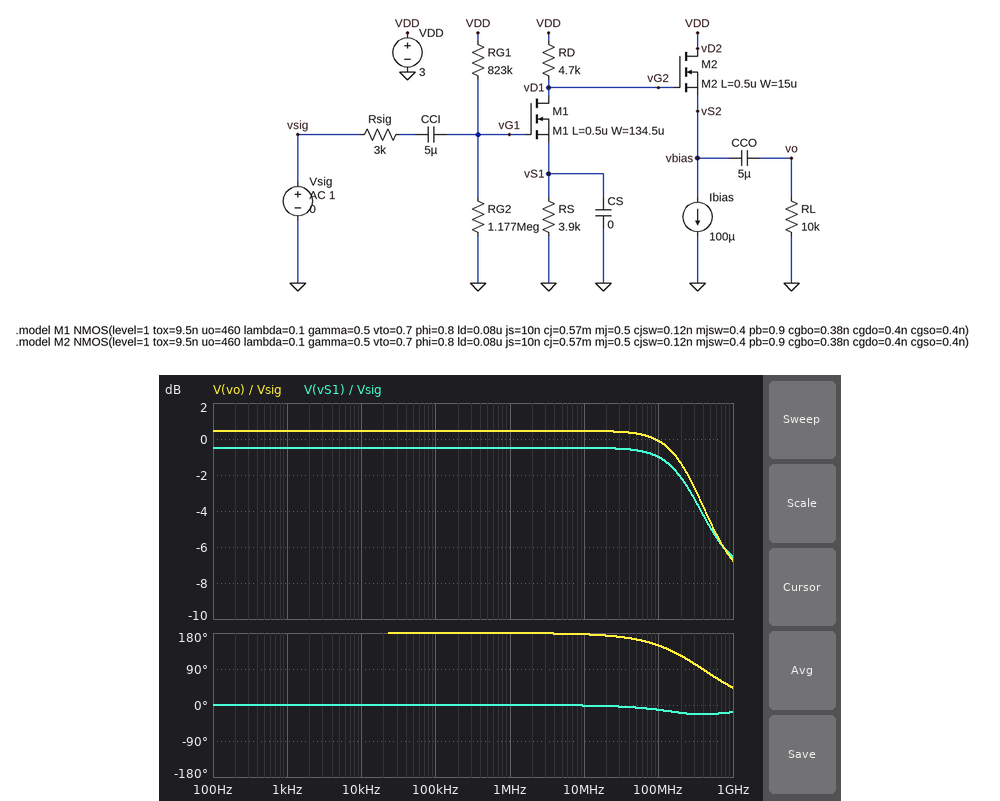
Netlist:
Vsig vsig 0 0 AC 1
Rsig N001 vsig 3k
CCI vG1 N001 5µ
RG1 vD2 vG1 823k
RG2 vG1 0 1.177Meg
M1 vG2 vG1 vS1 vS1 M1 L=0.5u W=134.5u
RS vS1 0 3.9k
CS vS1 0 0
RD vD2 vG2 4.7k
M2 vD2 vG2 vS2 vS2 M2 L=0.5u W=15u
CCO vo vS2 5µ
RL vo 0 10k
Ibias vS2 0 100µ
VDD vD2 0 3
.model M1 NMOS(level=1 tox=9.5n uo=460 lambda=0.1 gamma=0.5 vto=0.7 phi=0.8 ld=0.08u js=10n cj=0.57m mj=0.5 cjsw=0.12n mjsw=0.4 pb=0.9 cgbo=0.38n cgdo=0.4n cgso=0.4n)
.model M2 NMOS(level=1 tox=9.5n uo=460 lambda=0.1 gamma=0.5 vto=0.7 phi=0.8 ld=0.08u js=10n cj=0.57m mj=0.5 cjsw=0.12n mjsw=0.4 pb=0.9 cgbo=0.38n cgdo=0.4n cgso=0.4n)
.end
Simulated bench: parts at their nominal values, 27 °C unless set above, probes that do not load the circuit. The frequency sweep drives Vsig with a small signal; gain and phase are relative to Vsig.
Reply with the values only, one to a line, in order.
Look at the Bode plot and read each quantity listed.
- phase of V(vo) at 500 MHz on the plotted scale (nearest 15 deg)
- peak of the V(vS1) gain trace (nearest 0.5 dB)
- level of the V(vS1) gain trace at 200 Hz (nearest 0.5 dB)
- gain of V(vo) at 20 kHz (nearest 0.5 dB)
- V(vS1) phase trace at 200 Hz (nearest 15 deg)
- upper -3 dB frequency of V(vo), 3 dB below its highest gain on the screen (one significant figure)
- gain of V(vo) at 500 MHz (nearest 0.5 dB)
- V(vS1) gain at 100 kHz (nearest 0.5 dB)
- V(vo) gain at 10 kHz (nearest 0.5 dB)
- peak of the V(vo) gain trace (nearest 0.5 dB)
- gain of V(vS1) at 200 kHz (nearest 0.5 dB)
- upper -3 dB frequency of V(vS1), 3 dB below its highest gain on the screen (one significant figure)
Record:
75 deg
-0.5 dB
-0.5 dB
0.5 dB
0 deg
300 MHz
-4.5 dB
-0.5 dB
0.5 dB
0.5 dB
-0.5 dB
300 MHz
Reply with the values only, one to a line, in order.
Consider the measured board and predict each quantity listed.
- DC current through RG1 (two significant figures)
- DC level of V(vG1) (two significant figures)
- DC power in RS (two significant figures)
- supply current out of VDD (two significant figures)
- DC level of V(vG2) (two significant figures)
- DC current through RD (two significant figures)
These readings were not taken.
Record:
1.5 µA
1.8 V
250 µW
350 µA
1.8 V
250 µA
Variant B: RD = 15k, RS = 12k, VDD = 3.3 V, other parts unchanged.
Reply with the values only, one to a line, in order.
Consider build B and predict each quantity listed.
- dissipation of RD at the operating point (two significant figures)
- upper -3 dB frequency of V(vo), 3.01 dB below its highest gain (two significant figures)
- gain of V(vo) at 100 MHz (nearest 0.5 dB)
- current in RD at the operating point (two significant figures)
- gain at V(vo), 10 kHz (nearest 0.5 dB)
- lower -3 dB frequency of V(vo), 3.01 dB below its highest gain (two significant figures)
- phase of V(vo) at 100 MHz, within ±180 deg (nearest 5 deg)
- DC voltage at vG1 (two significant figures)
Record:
150 µW
200 MHz
-0.5 dB
99 µA
1.0 dB
3.0 Hz
115 deg
1.9 V
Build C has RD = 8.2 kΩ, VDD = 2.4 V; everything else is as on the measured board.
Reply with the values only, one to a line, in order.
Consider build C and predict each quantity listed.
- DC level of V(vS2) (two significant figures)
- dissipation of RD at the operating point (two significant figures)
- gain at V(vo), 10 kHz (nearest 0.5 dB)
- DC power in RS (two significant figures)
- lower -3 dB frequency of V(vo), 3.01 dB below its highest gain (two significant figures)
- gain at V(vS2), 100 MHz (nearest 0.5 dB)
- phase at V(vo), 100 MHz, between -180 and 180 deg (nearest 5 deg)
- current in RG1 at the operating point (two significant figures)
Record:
200 mV
220 µW
5.0 dB
110 µW
3.0 Hz
4.0 dB
140 deg
1.2 µA
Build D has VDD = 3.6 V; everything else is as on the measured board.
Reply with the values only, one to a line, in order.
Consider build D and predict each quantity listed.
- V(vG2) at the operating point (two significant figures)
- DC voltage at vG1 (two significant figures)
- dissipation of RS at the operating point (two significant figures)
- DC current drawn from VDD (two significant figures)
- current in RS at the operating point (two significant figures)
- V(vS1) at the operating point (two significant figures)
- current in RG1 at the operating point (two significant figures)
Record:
2.0 V
2.1 V
450 µW
440 µA
340 µA
1.3 V
1.8 µA
